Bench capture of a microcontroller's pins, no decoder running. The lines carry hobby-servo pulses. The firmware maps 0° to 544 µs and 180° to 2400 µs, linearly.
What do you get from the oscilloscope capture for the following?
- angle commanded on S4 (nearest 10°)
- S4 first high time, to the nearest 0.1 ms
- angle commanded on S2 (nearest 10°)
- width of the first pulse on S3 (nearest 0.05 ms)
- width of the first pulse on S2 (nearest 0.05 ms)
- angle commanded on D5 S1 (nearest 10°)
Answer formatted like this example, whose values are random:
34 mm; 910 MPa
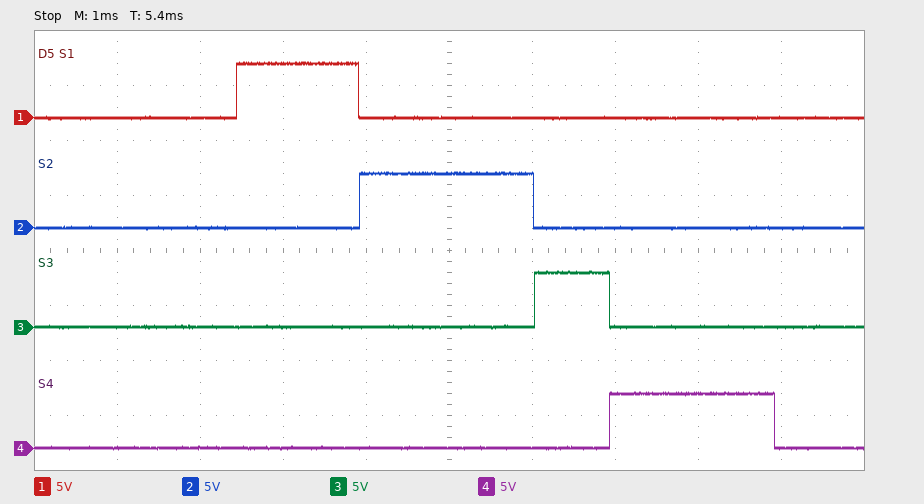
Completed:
140°; 2.0 ms; 150°; 0.90 ms; 2.10 ms; 90°
